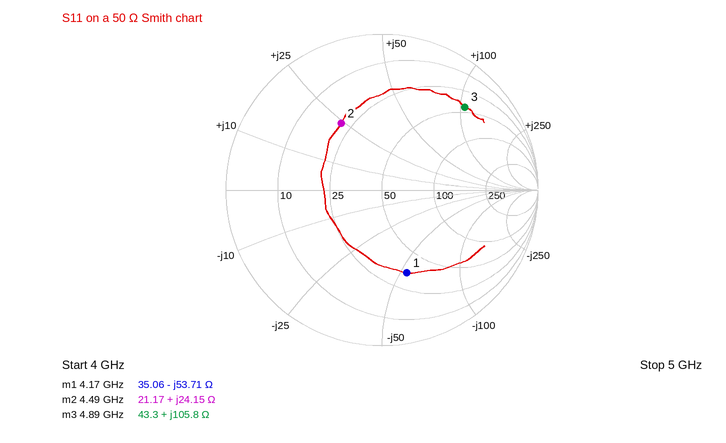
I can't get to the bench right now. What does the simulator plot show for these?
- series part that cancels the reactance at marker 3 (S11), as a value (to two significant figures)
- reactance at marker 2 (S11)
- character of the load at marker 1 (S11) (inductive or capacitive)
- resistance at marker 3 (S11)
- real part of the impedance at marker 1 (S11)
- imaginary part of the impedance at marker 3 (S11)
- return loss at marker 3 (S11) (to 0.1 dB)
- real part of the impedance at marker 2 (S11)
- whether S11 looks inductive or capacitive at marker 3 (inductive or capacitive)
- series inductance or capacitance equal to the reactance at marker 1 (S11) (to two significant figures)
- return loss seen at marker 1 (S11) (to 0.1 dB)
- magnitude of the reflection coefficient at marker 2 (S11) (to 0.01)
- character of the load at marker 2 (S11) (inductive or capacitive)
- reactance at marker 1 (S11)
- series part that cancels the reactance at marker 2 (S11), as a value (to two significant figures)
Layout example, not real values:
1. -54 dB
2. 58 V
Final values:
1. 310 fF
2. +24.15 Ω
3. capacitive
4. 43.3 Ω
5. 35.06 Ω
6. +105.8 Ω
7. 2.5 dB
8. 21.17 Ω
9. inductive
10. 710 fF
11. 5.1 dB
12. 0.50
13. inductive
14. -53.71 Ω
15. 1.5 pF
